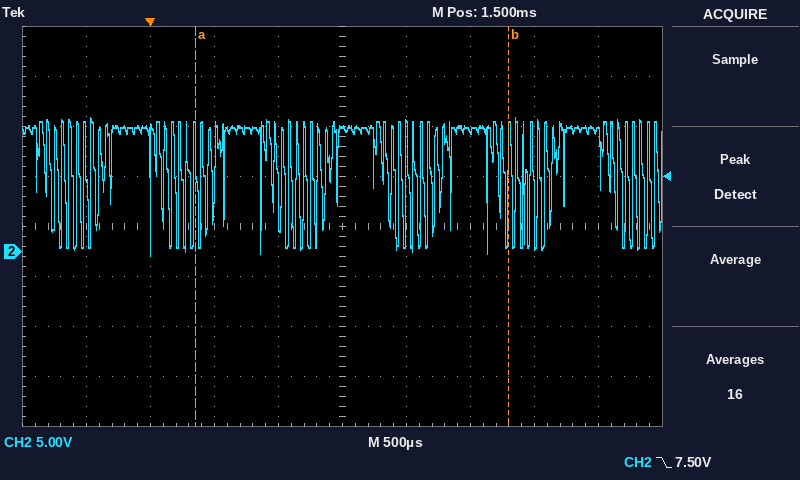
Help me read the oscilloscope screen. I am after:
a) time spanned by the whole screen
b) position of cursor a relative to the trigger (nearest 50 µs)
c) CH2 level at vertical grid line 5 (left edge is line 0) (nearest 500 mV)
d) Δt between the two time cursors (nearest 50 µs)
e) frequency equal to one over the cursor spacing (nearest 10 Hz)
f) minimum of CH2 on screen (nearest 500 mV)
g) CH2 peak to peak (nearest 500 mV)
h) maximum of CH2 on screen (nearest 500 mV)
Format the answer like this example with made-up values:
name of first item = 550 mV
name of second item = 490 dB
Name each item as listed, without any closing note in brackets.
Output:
time spanned by the whole screen = 5 ms
position of cursor a relative to the trigger = +350 µs
CH2 level at vertical grid line 5 (left edge is line 0) = 12.5 V
Δt between the two time cursors = 2.45 ms
frequency equal to one over the cursor spacing = 410 Hz
minimum of CH2 on screen = -500 mV
CH2 peak to peak = 14.0 V
maximum of CH2 on screen = 13.5 V
